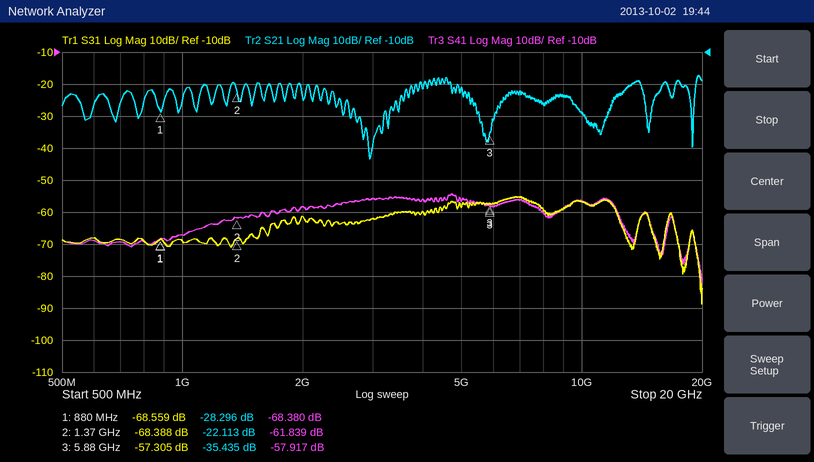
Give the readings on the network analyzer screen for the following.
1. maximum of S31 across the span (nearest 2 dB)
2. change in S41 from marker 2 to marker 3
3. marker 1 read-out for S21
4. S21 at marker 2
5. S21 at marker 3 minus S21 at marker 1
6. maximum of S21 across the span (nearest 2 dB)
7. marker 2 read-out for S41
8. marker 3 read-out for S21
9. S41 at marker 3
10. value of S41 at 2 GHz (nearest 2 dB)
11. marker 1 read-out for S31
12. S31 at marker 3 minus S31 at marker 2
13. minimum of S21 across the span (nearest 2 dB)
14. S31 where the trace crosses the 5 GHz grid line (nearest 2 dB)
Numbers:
-56 dB
3.922 dB
-28.296 dB
-22.113 dB
-7.139 dB
-18 dB
-61.839 dB
-35.435 dB
-57.917 dB
-58 dB
-68.559 dB
11.083 dB
-44 dB
-58 dB
